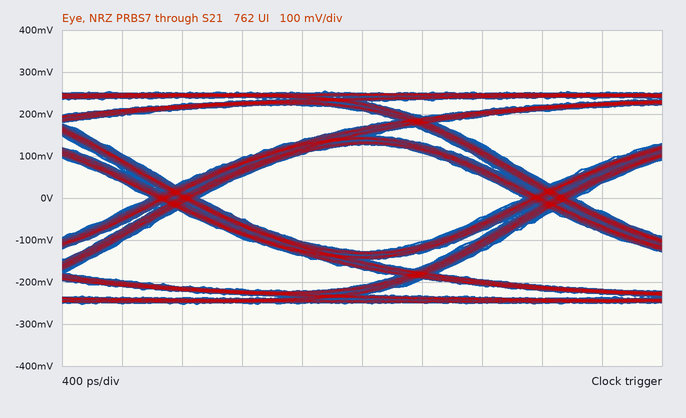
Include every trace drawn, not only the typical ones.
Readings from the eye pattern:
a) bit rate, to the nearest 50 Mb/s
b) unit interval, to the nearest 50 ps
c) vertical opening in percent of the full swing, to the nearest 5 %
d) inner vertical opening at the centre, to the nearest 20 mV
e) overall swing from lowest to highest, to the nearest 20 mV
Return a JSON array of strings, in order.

["400 Mb/s", "2.50 ns", "50 %", "260 mV", "500 mV"]
